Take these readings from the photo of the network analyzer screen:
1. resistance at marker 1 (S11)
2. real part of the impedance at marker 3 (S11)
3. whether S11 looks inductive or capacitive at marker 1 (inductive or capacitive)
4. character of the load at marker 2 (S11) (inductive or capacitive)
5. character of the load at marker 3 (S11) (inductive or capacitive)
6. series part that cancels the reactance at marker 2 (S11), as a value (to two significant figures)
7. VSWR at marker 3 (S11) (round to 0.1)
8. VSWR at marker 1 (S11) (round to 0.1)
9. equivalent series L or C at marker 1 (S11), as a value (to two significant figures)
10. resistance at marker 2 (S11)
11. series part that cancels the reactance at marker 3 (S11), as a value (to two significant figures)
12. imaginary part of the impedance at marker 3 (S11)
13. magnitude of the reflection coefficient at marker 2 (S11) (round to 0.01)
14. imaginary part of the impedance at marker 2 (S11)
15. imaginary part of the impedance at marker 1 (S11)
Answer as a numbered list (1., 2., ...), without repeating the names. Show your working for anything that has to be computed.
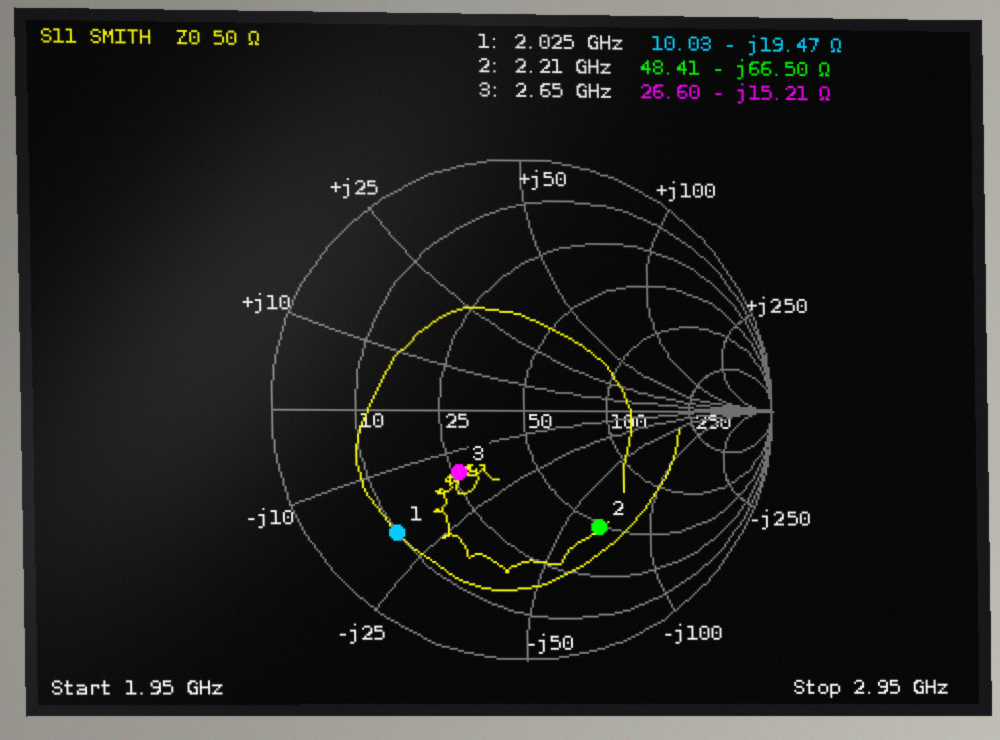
1. 10.03 Ω
2. 26.60 Ω
3. capacitive
4. capacitive
5. capacitive
6. L = 66.5 Ω/(2π × 2.21 GHz) ≈ 4.8 nH
7. 2.1
8. 5.8
9. C = 1/(2π × 2.025 GHz × 19.47 Ω) ≈ 4.0 pF
10. 48.41 Ω
11. L = 15.21 Ω/(2π × 2.65 GHz) ≈ 913 pH, so 910 pH to two significant figures
12. -15.21 Ω
13. 0.56
14. -66.50 Ω
15. -19.47 Ω
